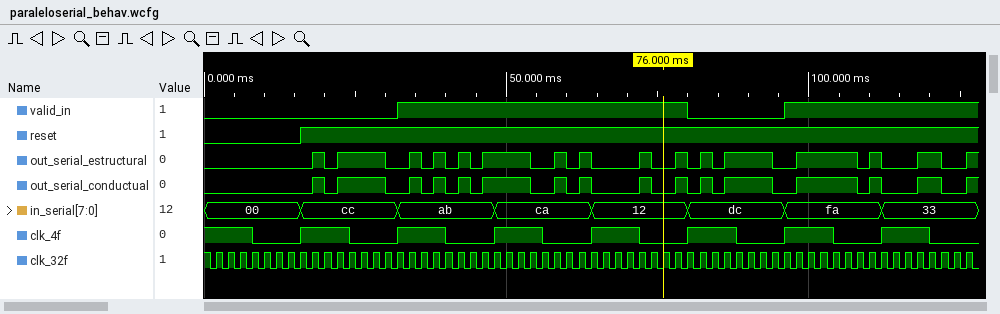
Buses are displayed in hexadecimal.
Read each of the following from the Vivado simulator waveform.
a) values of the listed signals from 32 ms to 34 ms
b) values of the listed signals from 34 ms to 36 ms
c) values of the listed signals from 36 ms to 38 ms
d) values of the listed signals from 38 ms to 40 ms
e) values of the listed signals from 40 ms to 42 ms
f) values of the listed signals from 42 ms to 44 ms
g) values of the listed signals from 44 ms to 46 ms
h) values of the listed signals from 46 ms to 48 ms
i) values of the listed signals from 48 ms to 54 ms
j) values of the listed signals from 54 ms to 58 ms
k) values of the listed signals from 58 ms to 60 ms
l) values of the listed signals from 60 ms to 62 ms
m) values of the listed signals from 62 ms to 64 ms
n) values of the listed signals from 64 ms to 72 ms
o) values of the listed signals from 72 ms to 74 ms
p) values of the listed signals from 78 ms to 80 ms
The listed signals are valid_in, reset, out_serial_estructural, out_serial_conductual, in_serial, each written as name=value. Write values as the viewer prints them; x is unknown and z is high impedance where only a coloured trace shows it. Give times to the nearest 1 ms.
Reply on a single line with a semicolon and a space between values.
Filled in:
valid_in=1, reset=1, out_serial_estructural=0, out_serial_conductual=0, in_serial=ab; valid_in=1, reset=1, out_serial_estructural=1, out_serial_conductual=1, in_serial=ab; valid_in=1, reset=1, out_serial_estructural=0, out_serial_conductual=0, in_serial=ab; valid_in=1, reset=1, out_serial_estructural=1, out_serial_conductual=1, in_serial=ab; valid_in=1, reset=1, out_serial_estructural=0, out_serial_conductual=0, in_serial=ab; valid_in=1, reset=1, out_serial_estructural=1, out_serial_conductual=1, in_serial=ab; valid_in=1, reset=1, out_serial_estructural=0, out_serial_conductual=0, in_serial=ab; valid_in=1, reset=1, out_serial_estructural=1, out_serial_conductual=1, in_serial=ab; valid_in=1, reset=1, out_serial_estructural=1, out_serial_conductual=1, in_serial=ca; valid_in=1, reset=1, out_serial_estructural=0, out_serial_conductual=0, in_serial=ca; valid_in=1, reset=1, out_serial_estructural=1, out_serial_conductual=1, in_serial=ca; valid_in=1, reset=1, out_serial_estructural=0, out_serial_conductual=0, in_serial=ca; valid_in=1, reset=1, out_serial_estructural=1, out_serial_conductual=1, in_serial=ca; valid_in=1, reset=1, out_serial_estructural=0, out_serial_conductual=0, in_serial=12; valid_in=1, reset=1, out_serial_estructural=1, out_serial_conductual=1, in_serial=12; valid_in=1, reset=1, out_serial_estructural=1, out_serial_conductual=1, in_serial=12
